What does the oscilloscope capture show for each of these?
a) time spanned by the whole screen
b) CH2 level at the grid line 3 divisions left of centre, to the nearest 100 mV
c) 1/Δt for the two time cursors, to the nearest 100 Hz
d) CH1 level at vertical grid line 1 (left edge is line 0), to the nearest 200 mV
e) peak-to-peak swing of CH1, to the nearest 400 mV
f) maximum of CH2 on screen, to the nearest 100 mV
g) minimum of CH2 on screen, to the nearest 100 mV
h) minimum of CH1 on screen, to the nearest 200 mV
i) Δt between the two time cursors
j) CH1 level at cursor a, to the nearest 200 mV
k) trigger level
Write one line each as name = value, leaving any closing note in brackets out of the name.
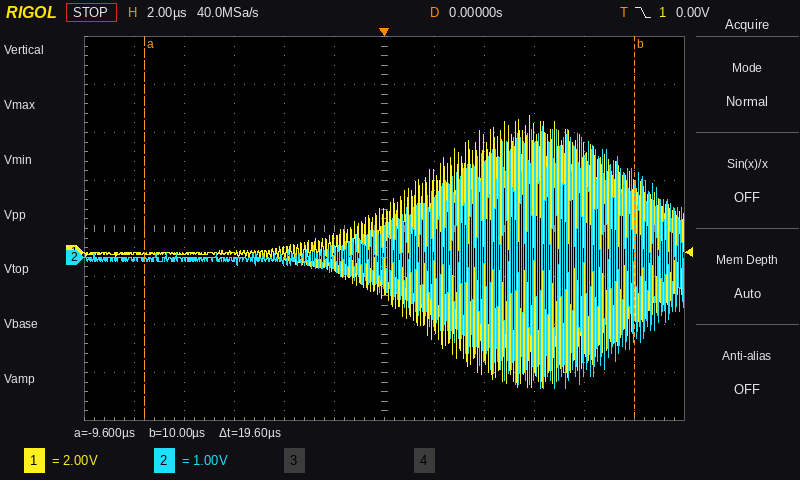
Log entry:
time spanned by the whole screen = 24 µs
CH2 level at the grid line 3 divisions left of centre, to the nearest 100 mV = -100 mV
1/Δt for the two time cursors, to the nearest 100 Hz = 51.0 kHz
CH1 level at vertical grid line 1 (left edge is line 0), to the nearest 200 mV = 0.0 V
peak-to-peak swing of CH1, to the nearest 400 mV = 11.2 V
maximum of CH2 on screen, to the nearest 100 mV = 2.7 V
minimum of CH2 on screen, to the nearest 100 mV = -2.7 V
minimum of CH1 on screen, to the nearest 200 mV = -5.6 V
Δt between the two time cursors = 19.6 µs
CH1 level at cursor a, to the nearest 200 mV = 0.0 V
trigger level = 0.00 V
